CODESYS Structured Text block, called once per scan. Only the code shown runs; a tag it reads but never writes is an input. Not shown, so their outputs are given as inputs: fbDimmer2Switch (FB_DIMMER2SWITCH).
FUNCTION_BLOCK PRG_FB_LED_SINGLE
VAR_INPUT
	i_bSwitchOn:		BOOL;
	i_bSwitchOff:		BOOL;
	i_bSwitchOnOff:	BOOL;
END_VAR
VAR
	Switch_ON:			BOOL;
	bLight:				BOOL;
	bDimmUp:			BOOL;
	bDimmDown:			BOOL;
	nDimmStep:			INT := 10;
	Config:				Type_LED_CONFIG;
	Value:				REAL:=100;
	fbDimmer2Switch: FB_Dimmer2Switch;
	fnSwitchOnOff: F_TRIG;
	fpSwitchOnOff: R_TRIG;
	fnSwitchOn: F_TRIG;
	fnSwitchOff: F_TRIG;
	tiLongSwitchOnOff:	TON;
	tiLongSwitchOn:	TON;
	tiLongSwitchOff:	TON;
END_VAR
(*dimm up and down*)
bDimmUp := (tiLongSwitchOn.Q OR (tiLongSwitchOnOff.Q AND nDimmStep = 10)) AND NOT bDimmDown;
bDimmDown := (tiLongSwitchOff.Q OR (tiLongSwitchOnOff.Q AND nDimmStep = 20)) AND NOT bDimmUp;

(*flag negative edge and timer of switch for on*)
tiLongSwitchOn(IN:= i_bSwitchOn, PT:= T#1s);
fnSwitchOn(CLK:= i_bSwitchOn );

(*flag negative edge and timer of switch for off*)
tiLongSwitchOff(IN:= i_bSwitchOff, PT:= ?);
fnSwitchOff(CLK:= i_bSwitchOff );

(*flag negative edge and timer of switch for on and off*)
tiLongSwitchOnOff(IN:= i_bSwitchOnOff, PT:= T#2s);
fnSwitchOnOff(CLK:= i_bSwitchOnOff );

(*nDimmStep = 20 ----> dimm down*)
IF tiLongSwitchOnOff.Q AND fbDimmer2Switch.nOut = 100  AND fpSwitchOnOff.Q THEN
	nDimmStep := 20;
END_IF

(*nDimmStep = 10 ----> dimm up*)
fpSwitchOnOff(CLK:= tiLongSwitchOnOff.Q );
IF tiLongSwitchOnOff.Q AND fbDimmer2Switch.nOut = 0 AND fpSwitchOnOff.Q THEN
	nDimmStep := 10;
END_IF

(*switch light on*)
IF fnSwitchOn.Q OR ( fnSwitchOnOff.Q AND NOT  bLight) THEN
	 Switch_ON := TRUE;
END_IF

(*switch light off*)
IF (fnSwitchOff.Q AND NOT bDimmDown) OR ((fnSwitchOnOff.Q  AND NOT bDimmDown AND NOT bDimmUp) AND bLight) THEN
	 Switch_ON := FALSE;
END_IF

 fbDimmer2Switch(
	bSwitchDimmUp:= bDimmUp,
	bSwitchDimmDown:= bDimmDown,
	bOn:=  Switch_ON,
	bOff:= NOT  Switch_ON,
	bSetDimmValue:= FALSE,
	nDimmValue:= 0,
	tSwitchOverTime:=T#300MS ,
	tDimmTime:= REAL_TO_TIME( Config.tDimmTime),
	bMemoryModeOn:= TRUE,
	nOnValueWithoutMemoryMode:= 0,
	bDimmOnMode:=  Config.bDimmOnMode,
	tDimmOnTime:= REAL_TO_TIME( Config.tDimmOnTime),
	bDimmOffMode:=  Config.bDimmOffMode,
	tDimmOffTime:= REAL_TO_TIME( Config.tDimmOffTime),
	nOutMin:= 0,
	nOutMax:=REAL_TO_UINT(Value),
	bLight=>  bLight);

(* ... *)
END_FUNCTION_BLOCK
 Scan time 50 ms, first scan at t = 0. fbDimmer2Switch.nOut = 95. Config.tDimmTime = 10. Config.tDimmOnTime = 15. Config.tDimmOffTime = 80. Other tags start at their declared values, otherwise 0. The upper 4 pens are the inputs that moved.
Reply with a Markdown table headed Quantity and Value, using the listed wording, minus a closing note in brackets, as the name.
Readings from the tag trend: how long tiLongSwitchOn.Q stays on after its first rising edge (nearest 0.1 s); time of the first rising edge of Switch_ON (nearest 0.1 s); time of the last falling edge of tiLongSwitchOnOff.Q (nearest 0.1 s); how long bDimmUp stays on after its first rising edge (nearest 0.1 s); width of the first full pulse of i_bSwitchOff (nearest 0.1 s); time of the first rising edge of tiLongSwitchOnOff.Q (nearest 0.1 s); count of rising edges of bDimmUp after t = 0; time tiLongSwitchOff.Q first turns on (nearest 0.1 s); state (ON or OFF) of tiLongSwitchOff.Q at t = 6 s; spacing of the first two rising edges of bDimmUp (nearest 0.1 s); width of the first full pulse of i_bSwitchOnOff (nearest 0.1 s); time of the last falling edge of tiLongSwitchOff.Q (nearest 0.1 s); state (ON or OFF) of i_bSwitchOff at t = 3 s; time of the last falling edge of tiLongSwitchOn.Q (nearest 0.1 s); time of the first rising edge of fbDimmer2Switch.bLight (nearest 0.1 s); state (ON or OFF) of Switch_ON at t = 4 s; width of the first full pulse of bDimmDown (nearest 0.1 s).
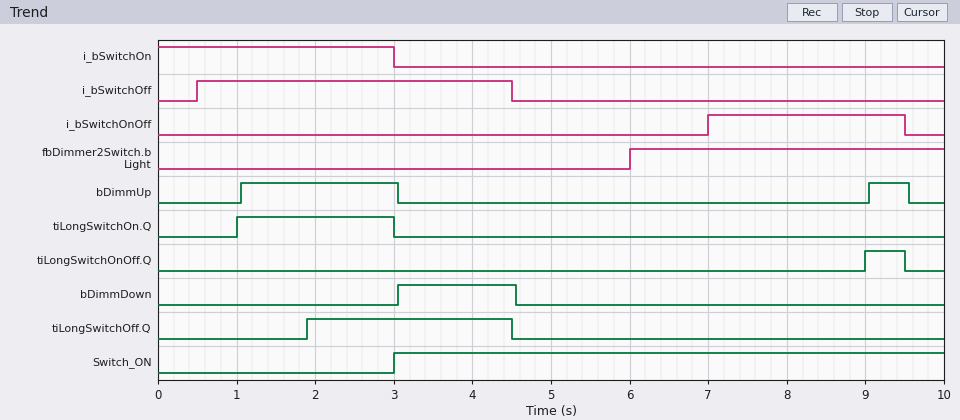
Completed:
| Quantity | Value |
|---|---|
| how long tiLongSwitchOn.Q stays on after its first rising edge | 2.0 s |
| time of the first rising edge of Switch_ON | 3.0 s |
| time of the last falling edge of tiLongSwitchOnOff.Q | 9.5 s |
| how long bDimmUp stays on after its first rising edge | 2.0 s |
| width of the first full pulse of i_bSwitchOff | 4.0 s |
| time of the first rising edge of tiLongSwitchOnOff.Q | 9.0 s |
| count of rising edges of bDimmUp after t = 0 | 2 |
| time tiLongSwitchOff.Q first turns on | 1.9 s |
| state (ON or OFF) of tiLongSwitchOff.Q at t = 6 s | OFF |
| spacing of the first two rising edges of bDimmUp | 8.0 s |
| width of the first full pulse of i_bSwitchOnOff | 2.5 s |
| time of the last falling edge of tiLongSwitchOff.Q | 4.5 s |
| state (ON or OFF) of i_bSwitchOff at t = 3 s | ON |
| time of the last falling edge of tiLongSwitchOn.Q | 3.0 s |
| time of the first rising edge of fbDimmer2Switch.bLight | 6.0 s |
| state (ON or OFF) of Switch_ON at t = 4 s | ON |
| width of the first full pulse of bDimmDown | 1.5 s |
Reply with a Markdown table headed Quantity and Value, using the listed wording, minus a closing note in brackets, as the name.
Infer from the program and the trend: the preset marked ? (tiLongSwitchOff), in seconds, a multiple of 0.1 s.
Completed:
| Quantity | Value |
|---|---|
| the preset marked ? (tiLongSwitchOff), in seconds, a multiple of 0.1 s | 1.4 s |
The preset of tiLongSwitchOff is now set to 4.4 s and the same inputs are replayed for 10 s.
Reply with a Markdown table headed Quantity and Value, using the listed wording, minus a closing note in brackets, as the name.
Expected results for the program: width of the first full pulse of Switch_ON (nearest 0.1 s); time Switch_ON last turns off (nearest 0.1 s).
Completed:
| Quantity | Value |
|---|---|
| width of the first full pulse of Switch_ON | 1.5 s |
| time Switch_ON last turns off | 4.5 s |
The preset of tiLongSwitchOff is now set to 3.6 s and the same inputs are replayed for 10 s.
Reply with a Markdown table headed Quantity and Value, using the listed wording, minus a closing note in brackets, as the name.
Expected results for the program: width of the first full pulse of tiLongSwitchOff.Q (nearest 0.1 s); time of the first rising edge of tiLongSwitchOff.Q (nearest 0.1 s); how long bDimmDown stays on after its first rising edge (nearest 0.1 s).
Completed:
| Quantity | Value |
|---|---|
| width of the first full pulse of tiLongSwitchOff.Q | 0.4 s |
| time of the first rising edge of tiLongSwitchOff.Q | 4.1 s |
| how long bDimmDown stays on after its first rising edge | 0.4 s |
